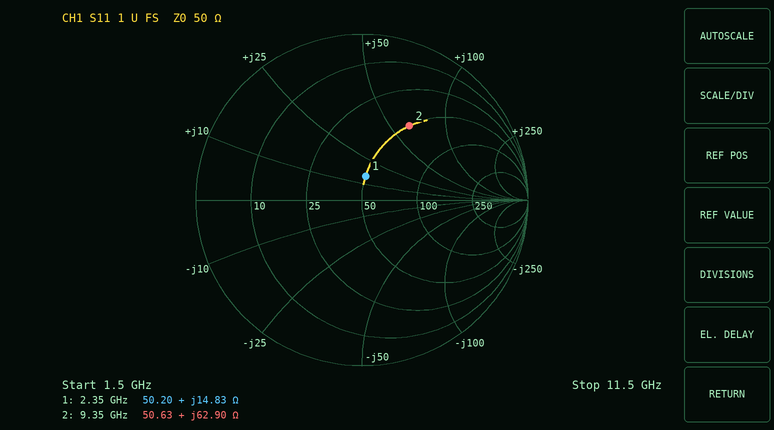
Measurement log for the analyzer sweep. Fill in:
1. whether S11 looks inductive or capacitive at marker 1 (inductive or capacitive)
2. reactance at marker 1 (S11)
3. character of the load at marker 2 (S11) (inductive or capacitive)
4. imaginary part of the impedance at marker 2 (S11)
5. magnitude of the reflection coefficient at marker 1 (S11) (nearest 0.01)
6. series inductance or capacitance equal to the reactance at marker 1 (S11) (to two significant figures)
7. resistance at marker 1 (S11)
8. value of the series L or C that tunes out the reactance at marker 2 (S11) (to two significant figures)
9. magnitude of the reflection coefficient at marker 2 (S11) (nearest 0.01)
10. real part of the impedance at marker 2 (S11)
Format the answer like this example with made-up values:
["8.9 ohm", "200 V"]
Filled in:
["inductive", "+14.83 Ω", "inductive", "+62.90 Ω", "0.15", "1.0 nH", "50.20 Ω", "270 fF", "0.53", "50.63 Ω"]
